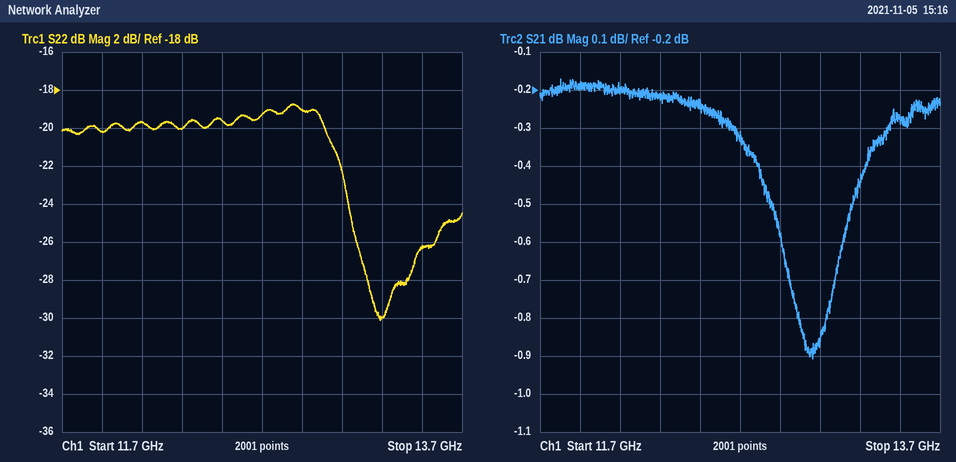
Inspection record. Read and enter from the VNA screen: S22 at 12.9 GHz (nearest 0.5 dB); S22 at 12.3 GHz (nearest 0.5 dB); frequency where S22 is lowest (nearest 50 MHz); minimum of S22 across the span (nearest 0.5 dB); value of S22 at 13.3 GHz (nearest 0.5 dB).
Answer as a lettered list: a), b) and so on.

a) -19.0 dB
b) -20.0 dB
c) 13.30 GHz
d) -30.0 dB
e) -30.0 dB
